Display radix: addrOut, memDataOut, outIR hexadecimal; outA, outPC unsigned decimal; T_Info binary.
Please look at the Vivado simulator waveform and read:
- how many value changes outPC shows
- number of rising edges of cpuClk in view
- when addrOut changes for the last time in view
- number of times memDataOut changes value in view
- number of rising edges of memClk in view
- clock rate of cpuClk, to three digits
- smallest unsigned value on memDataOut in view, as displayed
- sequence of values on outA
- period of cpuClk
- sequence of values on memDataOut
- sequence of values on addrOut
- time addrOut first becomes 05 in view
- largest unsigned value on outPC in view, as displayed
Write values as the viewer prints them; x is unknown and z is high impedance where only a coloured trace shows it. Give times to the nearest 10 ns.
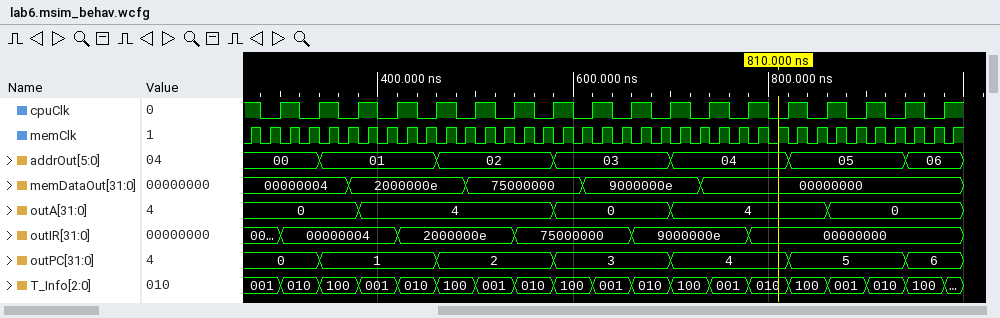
6
18
940 ns
4
37
25.0 MHz
00000000
0, 4, 0, 4, 0
40 ns
00000004, 2000000e, 75000000, 9000000e, 00000000
00, 01, 02, 03, 04, 05, 06
820 ns
6
